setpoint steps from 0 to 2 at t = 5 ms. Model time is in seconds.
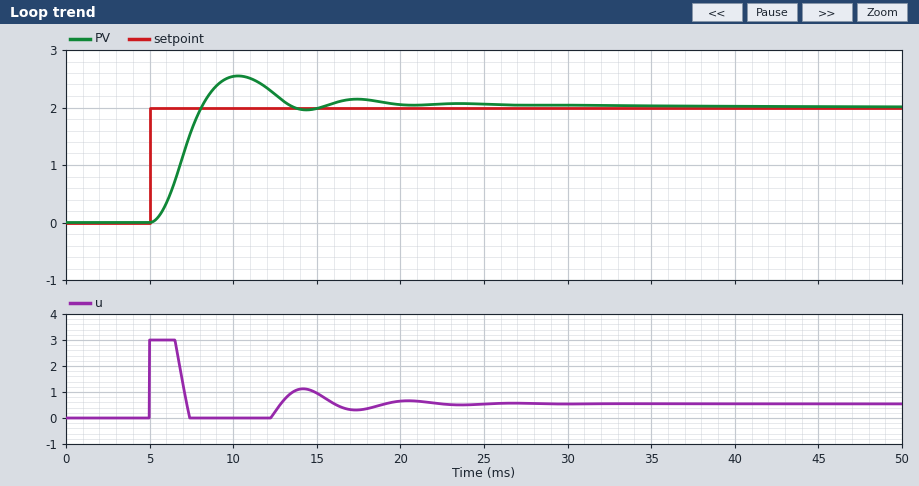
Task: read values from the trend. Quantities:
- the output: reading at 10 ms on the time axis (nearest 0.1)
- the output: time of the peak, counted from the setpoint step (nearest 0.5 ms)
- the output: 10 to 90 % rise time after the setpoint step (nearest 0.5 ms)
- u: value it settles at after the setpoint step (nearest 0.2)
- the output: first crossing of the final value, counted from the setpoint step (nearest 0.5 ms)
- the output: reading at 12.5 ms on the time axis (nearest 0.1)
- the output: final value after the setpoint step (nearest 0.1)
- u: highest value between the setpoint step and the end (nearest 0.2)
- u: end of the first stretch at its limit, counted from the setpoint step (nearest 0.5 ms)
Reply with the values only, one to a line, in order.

2.5
5.5 ms
2.0 ms
0.6
3.0 ms
2.2
2.0
3.0
1.5 ms
